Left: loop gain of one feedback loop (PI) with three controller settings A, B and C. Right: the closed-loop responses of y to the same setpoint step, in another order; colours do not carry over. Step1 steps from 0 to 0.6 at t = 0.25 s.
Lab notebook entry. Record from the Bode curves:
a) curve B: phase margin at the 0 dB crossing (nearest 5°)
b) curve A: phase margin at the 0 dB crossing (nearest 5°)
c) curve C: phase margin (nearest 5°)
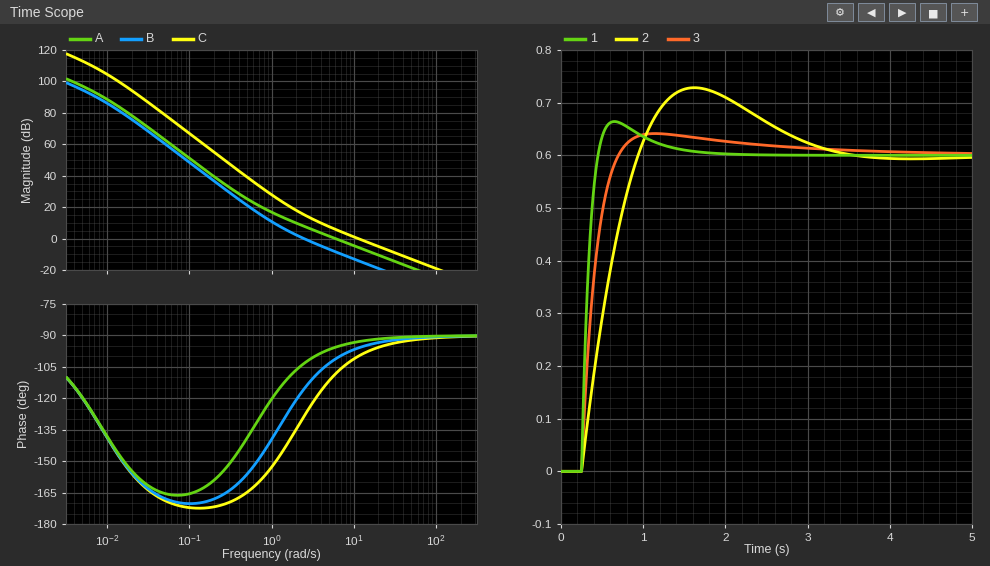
65°
85°
80°
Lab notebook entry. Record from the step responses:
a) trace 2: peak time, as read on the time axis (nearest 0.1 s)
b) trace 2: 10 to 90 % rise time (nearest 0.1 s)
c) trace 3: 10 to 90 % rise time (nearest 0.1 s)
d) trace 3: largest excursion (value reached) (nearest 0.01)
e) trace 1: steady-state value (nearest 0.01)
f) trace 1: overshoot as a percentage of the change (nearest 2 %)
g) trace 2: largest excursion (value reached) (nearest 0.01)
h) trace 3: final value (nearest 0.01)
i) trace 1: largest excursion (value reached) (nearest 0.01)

1.6 s
0.5 s
0.3 s
0.64
0.60
10 %
0.73
0.60
0.66
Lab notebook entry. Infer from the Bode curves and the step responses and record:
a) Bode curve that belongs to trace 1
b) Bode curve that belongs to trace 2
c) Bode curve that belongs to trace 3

C
B
A
